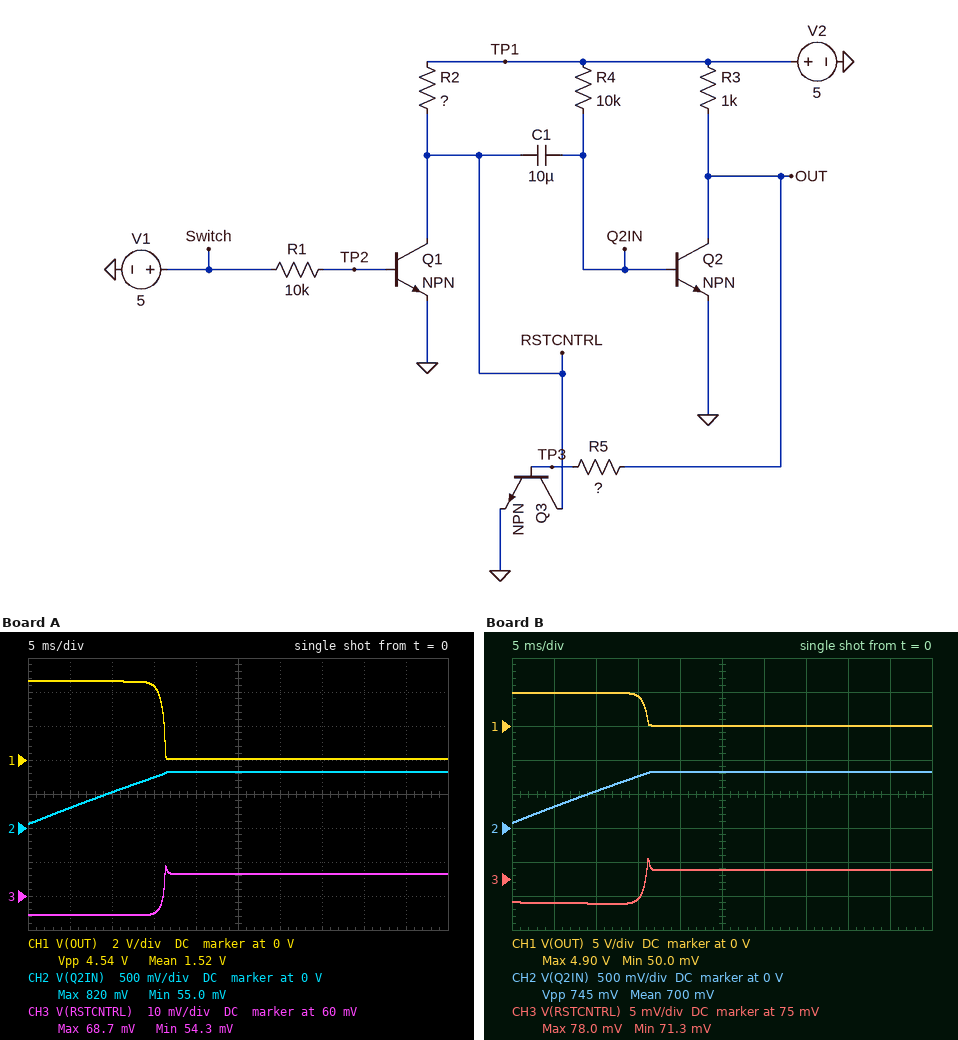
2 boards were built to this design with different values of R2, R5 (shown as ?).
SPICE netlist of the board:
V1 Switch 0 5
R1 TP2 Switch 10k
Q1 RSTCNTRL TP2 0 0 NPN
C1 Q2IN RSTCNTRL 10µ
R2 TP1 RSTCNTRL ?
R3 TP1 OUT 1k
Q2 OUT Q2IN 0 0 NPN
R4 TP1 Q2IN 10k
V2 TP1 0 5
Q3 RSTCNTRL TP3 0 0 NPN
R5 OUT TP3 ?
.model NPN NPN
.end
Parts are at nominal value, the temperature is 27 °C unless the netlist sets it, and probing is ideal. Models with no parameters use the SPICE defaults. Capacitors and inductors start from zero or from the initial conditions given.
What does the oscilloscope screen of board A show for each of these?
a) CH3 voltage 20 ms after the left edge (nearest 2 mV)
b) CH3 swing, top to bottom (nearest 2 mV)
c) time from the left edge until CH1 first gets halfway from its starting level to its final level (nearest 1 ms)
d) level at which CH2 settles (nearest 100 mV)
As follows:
66 mV
14 mV
16 ms
800 mV
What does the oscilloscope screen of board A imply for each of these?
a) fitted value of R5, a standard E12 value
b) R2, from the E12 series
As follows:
10 kΩ
1.2 kΩ
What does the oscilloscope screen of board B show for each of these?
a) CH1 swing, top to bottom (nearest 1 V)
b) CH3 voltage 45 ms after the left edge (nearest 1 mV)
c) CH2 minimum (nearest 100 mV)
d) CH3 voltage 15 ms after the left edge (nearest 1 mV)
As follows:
5 V
76 mV
100 mV
72 mV
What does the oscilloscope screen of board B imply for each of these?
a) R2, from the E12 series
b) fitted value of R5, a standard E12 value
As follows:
820 Ω
33 kΩ
